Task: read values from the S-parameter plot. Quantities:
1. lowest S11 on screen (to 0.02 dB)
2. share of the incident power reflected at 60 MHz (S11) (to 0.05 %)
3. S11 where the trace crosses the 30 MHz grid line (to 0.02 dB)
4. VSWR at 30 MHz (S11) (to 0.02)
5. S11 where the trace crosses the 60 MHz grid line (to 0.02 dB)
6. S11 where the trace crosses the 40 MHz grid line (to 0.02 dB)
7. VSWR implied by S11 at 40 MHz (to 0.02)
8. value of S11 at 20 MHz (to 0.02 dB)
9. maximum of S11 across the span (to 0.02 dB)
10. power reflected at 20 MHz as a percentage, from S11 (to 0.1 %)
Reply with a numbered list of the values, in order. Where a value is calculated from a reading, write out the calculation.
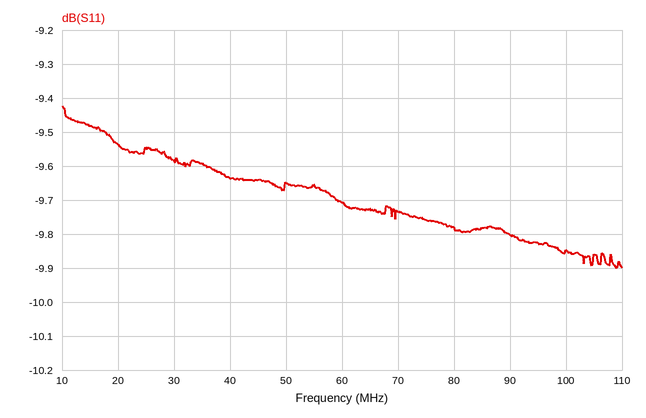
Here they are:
1. -9.90 dB
2. 10^(-9.7/10) ≈ 10.70 %
3. -9.58 dB
4. |Γ| = 10^(-9.58/20) = 0.3319; VSWR = (1 + 0.3319)/(1 − 0.3319) ≈ 1.99, so 2.00 to the nearest 0.02
5. -9.70 dB
6. -9.64 dB
7. |Γ| = 10^(-9.64/20) = 0.3296; VSWR = (1 + 0.3296)/(1 − 0.3296) ≈ 1.98
8. -9.54 dB
9. -9.42 dB
10. 10^(-9.54/10) ≈ 11.1 %
